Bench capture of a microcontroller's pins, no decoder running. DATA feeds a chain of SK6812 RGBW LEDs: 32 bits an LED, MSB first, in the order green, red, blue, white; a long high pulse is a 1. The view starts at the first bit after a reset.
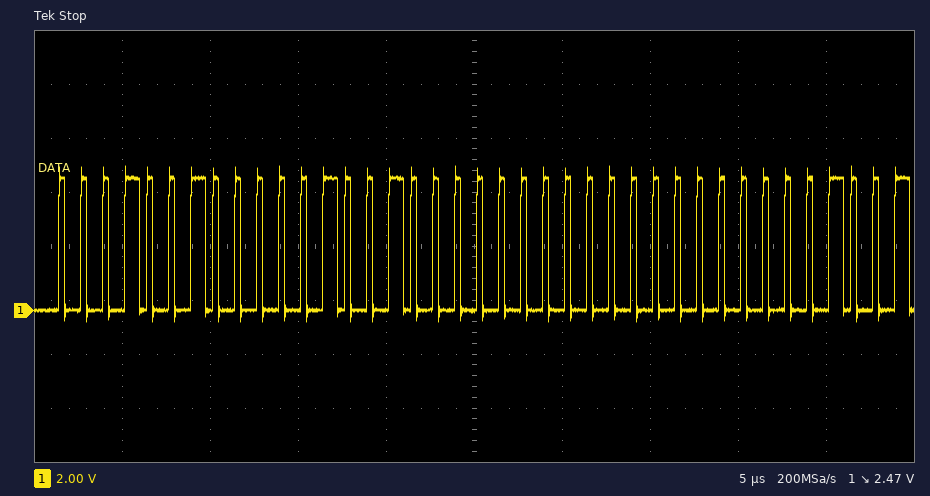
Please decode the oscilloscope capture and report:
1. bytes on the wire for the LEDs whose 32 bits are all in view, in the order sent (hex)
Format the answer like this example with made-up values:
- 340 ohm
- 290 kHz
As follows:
- 12 09 00 00
